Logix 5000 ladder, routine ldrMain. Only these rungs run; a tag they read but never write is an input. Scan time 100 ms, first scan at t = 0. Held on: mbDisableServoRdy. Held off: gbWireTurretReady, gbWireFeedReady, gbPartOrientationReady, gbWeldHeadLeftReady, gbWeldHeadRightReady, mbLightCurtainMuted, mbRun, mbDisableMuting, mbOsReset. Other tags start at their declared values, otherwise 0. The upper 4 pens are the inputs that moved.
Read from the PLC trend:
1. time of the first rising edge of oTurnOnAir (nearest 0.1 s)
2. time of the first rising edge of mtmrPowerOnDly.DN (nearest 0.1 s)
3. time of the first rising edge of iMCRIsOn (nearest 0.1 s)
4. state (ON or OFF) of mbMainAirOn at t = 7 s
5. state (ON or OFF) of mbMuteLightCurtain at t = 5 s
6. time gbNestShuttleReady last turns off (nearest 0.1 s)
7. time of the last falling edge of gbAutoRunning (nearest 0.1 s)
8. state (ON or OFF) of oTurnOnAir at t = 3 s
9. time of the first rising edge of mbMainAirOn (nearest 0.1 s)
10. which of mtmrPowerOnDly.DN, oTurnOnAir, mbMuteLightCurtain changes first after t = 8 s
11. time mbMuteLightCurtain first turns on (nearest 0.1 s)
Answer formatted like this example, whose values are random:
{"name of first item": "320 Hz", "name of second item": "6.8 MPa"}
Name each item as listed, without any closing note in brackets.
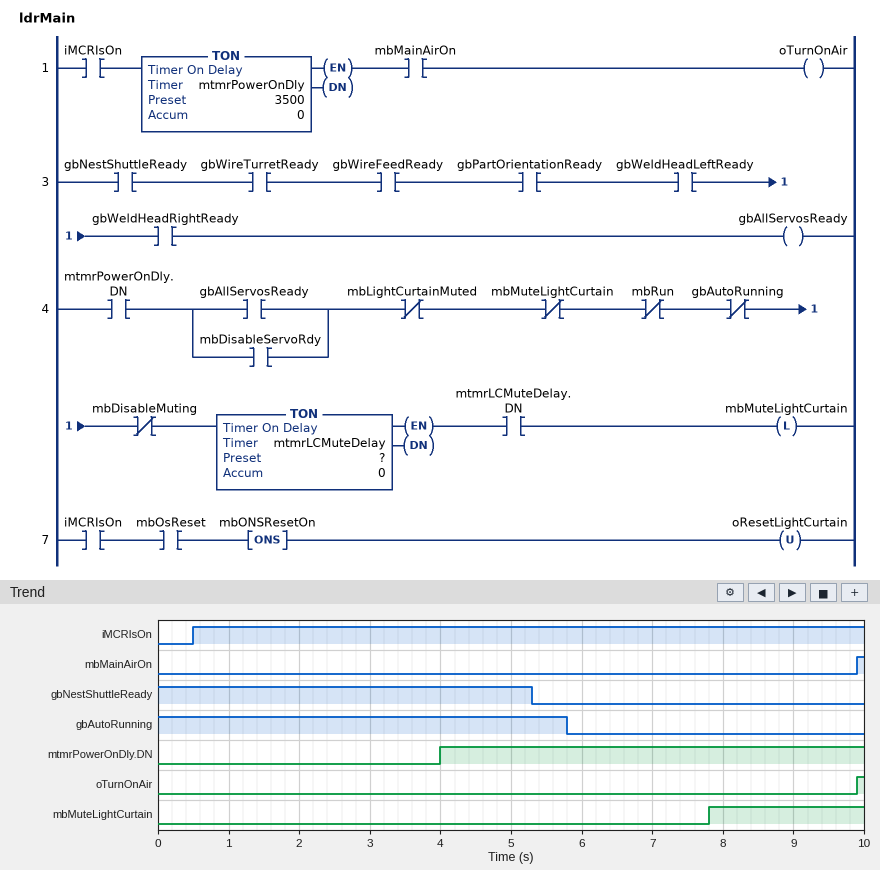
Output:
{"time of the first rising edge of oTurnOnAir": "9.9 s", "time of the first rising edge of mtmrPowerOnDly.DN": "4.0 s", "time of the first rising edge of iMCRIsOn": "0.5 s", "state (ON or OFF) of mbMainAirOn at t = 7 s": "OFF", "state (ON or OFF) of mbMuteLightCurtain at t = 5 s": "OFF", "time gbNestShuttleReady last turns off": "5.3 s", "time of the last falling edge of gbAutoRunning": "5.8 s", "state (ON or OFF) of oTurnOnAir at t = 3 s": "OFF", "time of the first rising edge of mbMainAirOn": "9.9 s", "which of mtmrPowerOnDly.DN, oTurnOnAir, mbMuteLightCurtain changes first after t = 8 s": "oTurnOnAir", "time mbMuteLightCurtain first turns on": "7.8 s"}
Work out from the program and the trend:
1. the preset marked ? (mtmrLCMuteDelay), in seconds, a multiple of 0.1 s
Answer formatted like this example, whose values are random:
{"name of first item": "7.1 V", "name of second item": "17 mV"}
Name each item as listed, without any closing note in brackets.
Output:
{"the preset marked ? (mtmrLCMuteDelay), in seconds, a multiple of 0.1 s": "2.0 s"}
